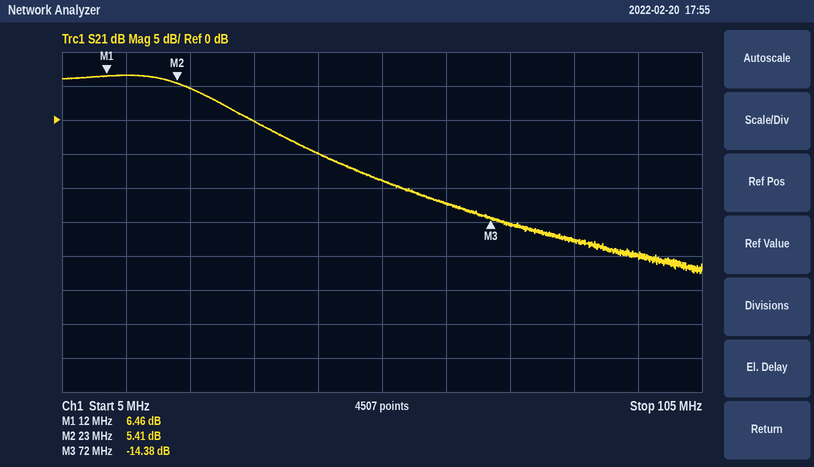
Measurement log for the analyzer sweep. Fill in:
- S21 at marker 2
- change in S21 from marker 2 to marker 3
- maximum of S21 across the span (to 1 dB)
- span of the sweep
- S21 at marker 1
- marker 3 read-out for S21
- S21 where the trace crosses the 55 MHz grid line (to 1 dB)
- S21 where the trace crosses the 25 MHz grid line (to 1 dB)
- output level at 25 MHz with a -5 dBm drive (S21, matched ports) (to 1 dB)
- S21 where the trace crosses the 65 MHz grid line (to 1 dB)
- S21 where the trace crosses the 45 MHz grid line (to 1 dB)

5.41 dB
-19.79 dB
7 dB
100 MHz
6.46 dB
-14.38 dB
-9 dB
5 dB
0 dBm
-12 dB
-5 dB
